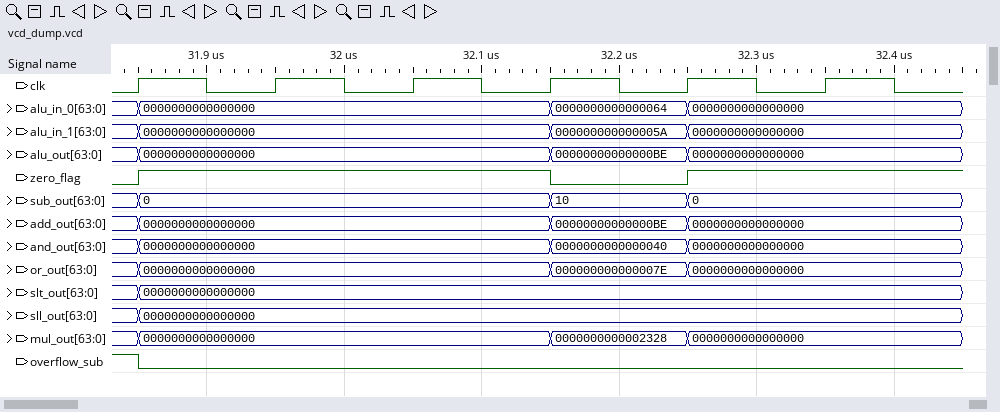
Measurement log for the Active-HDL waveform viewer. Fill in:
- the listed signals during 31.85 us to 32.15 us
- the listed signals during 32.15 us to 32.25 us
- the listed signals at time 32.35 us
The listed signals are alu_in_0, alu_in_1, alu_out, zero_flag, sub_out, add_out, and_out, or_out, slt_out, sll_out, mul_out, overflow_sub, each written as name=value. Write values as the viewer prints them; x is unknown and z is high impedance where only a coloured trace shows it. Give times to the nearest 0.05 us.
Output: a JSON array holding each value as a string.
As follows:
["alu_in_0=0000000000000000, alu_in_1=0000000000000000, alu_out=0000000000000000, zero_flag=1, sub_out=0, add_out=0000000000000000, and_out=0000000000000000, or_out=0000000000000000, slt_out=0000000000000000, sll_out=0000000000000000, mul_out=0000000000000000, overflow_sub=0", "alu_in_0=0000000000000064, alu_in_1=000000000000005A, alu_out=00000000000000BE, zero_flag=0, sub_out=10, add_out=00000000000000BE, and_out=0000000000000040, or_out=000000000000007E, slt_out=0000000000000000, sll_out=0000000000000000, mul_out=0000000000002328, overflow_sub=0", "alu_in_0=0000000000000000, alu_in_1=0000000000000000, alu_out=0000000000000000, zero_flag=1, sub_out=0, add_out=0000000000000000, and_out=0000000000000000, or_out=0000000000000000, slt_out=0000000000000000, sll_out=0000000000000000, mul_out=0000000000000000, overflow_sub=0"]
